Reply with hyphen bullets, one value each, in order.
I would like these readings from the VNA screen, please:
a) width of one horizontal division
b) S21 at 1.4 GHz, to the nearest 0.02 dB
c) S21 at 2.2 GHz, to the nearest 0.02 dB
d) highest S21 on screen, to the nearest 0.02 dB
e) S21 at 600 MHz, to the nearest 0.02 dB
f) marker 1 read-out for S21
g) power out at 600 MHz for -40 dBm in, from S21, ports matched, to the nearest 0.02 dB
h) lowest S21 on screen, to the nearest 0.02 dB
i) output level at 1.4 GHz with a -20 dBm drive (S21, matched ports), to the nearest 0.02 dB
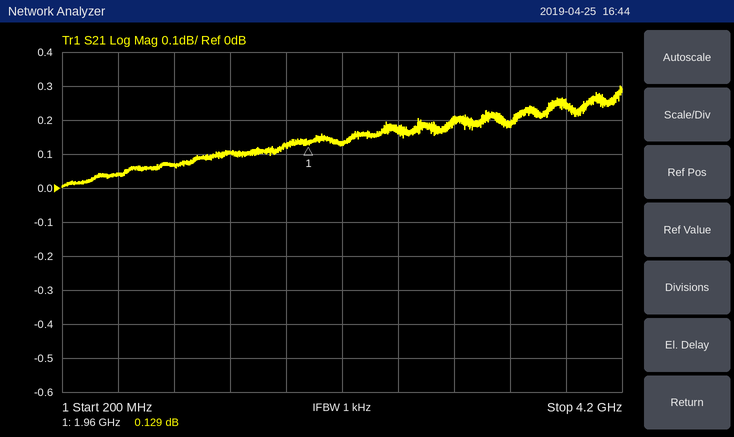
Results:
- 400 MHz
- 0.10 dB
- 0.14 dB
- 0.30 dB
- 0.04 dB
- 0.129 dB
- -39.96 dBm
- 0.00 dB
- -19.90 dBm
